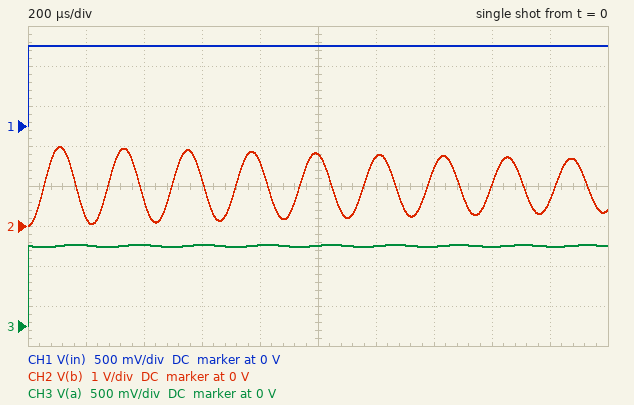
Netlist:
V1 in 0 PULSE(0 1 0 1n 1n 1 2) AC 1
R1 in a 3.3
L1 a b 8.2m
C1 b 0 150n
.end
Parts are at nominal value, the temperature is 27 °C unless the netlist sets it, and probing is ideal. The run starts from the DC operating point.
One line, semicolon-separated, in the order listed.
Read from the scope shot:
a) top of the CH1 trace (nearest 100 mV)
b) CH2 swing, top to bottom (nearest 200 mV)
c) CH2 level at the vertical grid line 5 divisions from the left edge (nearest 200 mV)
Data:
1.0 V; 2.0 V; 1.8 V
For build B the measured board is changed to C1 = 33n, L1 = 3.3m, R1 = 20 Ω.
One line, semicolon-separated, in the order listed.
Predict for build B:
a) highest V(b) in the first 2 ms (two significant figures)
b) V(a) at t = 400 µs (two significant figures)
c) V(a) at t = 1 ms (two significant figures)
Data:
1.9 V; 990 mV; 1.0 V
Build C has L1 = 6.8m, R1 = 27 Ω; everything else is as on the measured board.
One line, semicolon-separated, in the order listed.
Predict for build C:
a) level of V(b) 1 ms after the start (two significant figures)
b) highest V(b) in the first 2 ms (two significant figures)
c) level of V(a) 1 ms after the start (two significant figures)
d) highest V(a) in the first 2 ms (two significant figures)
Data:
870 mV; 1.8 V; 1.0 V; 1.1 V
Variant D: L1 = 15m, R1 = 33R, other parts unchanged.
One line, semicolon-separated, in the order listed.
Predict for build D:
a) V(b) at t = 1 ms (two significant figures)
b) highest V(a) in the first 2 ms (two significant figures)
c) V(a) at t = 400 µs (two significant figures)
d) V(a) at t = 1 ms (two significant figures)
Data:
1.2 V; 1.1 V; 940 mV; 970 mV
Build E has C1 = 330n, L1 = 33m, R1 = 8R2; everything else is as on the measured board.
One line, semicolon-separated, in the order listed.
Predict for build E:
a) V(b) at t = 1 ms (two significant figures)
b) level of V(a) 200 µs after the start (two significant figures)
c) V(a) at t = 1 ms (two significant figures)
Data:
1.9 V; 980 mV; 1.0 V
